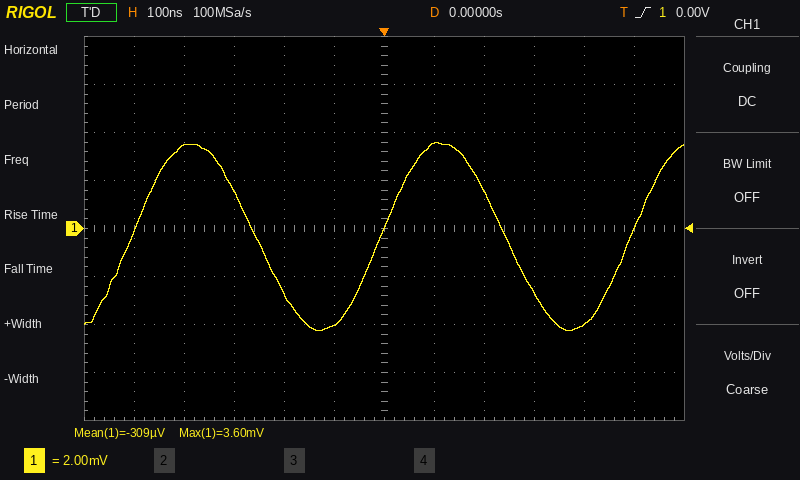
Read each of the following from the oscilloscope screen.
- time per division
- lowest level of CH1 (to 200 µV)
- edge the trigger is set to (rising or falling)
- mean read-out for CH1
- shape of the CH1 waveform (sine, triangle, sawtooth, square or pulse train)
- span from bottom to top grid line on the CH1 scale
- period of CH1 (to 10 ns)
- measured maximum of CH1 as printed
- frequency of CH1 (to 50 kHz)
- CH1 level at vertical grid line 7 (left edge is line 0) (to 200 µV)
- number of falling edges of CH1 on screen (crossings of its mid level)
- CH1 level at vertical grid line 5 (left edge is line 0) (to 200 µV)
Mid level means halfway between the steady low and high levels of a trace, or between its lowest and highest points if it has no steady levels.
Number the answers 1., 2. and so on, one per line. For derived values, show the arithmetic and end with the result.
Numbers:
1. 100 ns
2. -4.2 mV
3. rising
4. -309 µV
5. sine
6. 16 mV
7. 500 ns
8. 3.60 mV
9. 1 / 500 ns ≈ 2.00 MHz
10. 3.6 mV
11. 2
12. -4.0 mV
